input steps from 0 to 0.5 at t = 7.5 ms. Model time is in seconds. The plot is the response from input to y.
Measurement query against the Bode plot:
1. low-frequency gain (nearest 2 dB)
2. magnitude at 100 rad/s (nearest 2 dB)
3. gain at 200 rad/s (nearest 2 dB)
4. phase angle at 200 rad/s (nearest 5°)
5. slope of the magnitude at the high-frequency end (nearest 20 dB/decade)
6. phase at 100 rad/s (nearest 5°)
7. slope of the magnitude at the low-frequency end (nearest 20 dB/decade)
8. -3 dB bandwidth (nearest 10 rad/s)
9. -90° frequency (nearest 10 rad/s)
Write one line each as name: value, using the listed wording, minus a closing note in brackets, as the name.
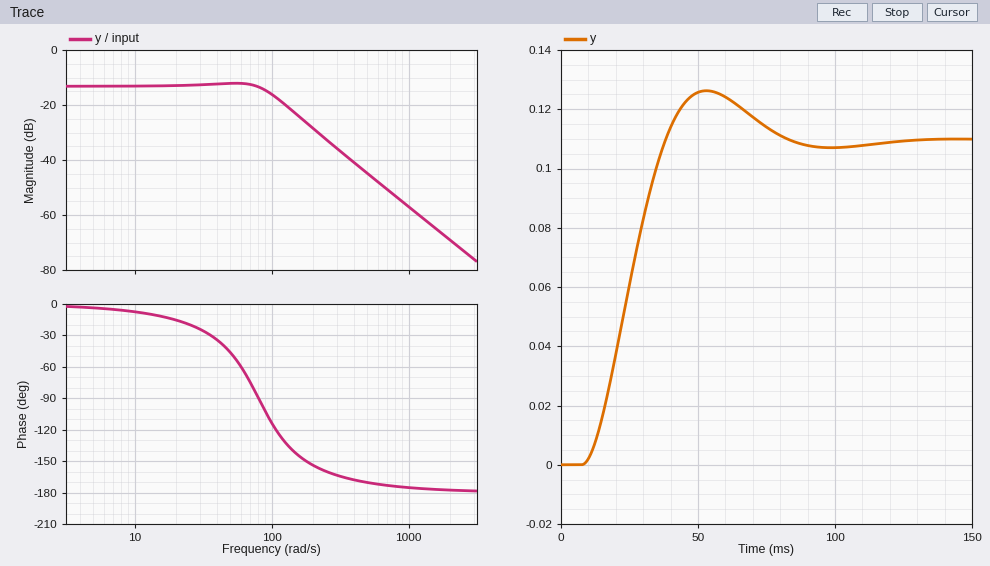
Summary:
low-frequency gain: -14 dB
magnitude at 100 rad/s: -16 dB
gain at 200 rad/s: -28 dB
phase angle at 200 rad/s: -155°
slope of the magnitude at the high-frequency end: -40 dB/decade
phase at 100 rad/s: -115°
slope of the magnitude at the low-frequency end: 0 dB/decade
-3 dB bandwidth: 100 rad/s
-90° frequency: 80 rad/s
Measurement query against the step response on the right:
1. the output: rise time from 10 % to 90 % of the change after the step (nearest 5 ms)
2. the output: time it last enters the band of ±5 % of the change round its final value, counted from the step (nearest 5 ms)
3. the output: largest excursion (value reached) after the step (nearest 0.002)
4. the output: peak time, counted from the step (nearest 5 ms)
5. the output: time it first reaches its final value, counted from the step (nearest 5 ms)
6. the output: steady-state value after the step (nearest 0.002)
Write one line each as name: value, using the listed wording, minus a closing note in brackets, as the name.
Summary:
the output: rise time from 10 % to 90 % of the change after the step: 20 ms
the output: time it last enters the band of ±5 % of the change round its final value, counted from the step: 65 ms
the output: largest excursion (value reached) after the step: 0.126
the output: peak time, counted from the step: 45 ms
the output: time it first reaches its final value, counted from the step: 30 ms
the output: steady-state value after the step: 0.110
